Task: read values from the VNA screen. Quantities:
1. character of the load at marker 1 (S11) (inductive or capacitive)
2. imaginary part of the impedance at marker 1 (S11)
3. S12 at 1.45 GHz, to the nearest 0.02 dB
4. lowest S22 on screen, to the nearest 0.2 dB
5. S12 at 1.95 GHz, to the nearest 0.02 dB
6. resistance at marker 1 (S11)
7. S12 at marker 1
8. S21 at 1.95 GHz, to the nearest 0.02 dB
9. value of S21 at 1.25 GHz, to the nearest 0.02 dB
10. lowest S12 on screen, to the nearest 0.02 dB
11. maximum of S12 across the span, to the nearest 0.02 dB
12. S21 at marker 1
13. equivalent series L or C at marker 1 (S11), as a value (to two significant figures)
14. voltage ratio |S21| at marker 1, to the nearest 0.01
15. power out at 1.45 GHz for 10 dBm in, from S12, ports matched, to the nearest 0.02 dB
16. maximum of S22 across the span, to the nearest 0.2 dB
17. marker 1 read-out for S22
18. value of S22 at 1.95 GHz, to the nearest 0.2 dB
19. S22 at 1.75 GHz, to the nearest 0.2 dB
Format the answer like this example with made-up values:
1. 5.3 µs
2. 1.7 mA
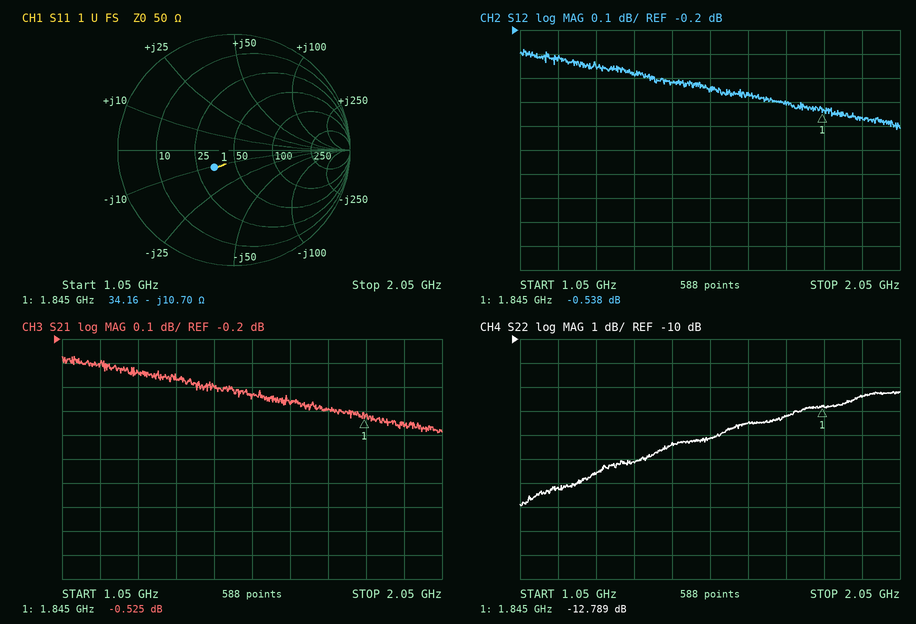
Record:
1. capacitive
2. -10.70 Ω
3. -0.42 dB
4. -17.0 dB
5. -0.56 dB
6. 34.16 Ω
7. -0.538 dB
8. -0.56 dB
9. -0.34 dB
10. -0.62 dB
11. -0.28 dB
12. -0.525 dB
13. 8.1 pF
14. 0.94
15. 9.58 dBm
16. -12.2 dB
17. -12.789 dB
18. -12.4 dB
19. -13.2 dB
